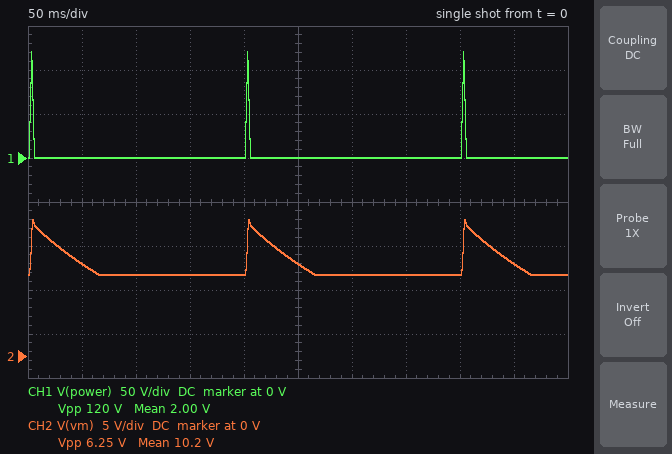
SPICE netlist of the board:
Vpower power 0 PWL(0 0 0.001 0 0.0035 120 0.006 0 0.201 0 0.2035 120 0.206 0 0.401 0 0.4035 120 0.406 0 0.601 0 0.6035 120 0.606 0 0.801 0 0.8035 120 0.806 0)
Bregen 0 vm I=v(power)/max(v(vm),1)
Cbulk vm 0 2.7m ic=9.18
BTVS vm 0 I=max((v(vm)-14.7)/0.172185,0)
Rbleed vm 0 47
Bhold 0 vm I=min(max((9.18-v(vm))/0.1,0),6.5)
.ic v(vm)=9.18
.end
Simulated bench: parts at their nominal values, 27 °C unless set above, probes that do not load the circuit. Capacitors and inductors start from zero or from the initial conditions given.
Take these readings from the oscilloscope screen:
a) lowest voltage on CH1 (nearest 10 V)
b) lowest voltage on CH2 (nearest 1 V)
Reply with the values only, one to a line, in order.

0 V
9 V
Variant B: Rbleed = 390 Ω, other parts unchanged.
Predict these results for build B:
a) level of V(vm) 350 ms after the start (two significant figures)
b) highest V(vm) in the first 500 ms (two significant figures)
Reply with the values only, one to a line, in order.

13 V
16 V
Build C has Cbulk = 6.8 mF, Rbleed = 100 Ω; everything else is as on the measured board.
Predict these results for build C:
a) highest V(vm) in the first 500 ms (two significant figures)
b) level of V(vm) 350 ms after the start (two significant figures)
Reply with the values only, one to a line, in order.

14 V
11 V
